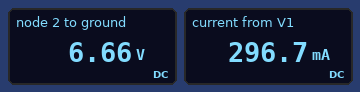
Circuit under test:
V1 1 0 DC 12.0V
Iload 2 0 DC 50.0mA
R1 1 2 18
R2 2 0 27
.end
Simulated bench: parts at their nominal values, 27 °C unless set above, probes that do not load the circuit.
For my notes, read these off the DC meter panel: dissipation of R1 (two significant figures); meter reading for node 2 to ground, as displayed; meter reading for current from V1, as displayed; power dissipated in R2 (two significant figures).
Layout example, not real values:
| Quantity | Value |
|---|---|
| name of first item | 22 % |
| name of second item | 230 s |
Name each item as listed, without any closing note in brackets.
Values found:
| Quantity | Value |
|---|---|
| dissipation of R1 | 1.6 W |
| meter reading for node 2 to ground, as displayed | 6.66 V |
| meter reading for current from V1, as displayed | 296.7 mA |
| power dissipated in R2 | 1.6 W |
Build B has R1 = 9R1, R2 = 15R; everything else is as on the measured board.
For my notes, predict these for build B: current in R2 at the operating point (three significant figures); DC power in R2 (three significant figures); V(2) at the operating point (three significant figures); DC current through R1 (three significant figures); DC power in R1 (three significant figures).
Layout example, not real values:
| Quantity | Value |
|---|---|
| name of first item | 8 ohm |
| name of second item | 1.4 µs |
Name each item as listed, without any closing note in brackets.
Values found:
| Quantity | Value |
|---|---|
| current in R2 at the operating point | 479 mA |
| DC power in R2 | 3.44 W |
| V(2) at the operating point | 7.19 V |
| DC current through R1 | 529 mA |
| DC power in R1 | 2.55 W |
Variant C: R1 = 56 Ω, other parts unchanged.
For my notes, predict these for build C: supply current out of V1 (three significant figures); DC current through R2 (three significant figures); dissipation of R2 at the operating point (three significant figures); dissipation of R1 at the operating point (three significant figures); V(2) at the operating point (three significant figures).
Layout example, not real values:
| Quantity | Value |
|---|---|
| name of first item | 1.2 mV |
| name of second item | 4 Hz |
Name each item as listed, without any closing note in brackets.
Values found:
| Quantity | Value |
|---|---|
| supply current out of V1 | 161 mA |
| DC current through R2 | 111 mA |
| dissipation of R2 at the operating point | 332 mW |
| dissipation of R1 at the operating point | 1.45 W |
| V(2) at the operating point | 2.99 V |
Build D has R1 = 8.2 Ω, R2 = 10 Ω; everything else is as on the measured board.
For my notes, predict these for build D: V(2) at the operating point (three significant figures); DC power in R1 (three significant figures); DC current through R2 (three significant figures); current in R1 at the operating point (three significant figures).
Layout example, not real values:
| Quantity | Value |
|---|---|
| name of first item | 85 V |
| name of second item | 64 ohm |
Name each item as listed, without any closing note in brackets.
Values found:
| Quantity | Value |
|---|---|
| V(2) at the operating point | 6.37 V |
| DC power in R1 | 3.87 W |
| DC current through R2 | 637 mA |
| current in R1 at the operating point | 687 mA |
